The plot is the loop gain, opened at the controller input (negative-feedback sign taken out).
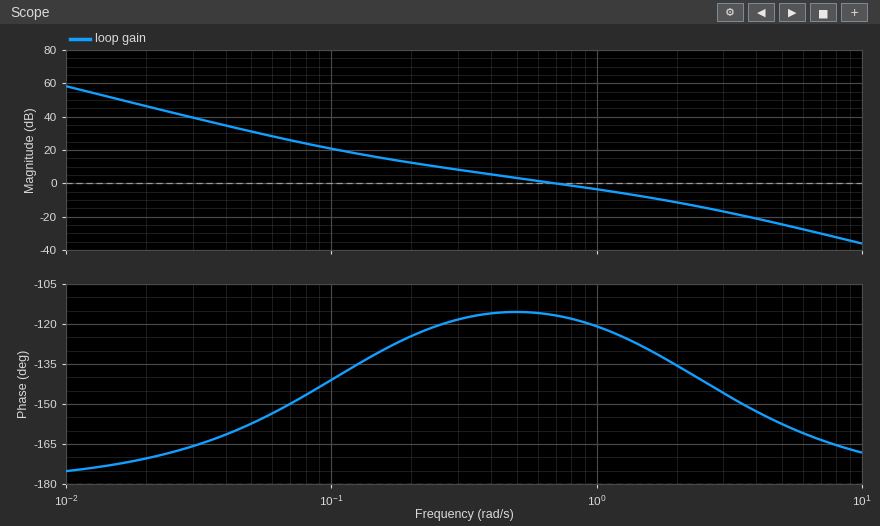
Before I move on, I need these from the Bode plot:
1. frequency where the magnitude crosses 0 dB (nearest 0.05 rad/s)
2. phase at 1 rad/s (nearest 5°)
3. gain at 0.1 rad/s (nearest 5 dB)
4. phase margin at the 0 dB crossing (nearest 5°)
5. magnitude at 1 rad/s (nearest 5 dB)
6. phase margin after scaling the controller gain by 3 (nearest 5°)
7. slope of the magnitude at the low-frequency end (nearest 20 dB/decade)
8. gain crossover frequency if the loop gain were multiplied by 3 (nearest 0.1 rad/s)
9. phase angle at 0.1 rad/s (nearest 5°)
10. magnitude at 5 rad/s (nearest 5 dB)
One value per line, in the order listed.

0.70 rad/s
-120°
20 dB
65°
-5 dB
50°
-40 dB/decade
1.7 rad/s
-140°
-25 dB
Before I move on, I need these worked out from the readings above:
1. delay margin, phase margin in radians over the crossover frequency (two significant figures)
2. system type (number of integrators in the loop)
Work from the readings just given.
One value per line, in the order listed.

1.6 s
2
